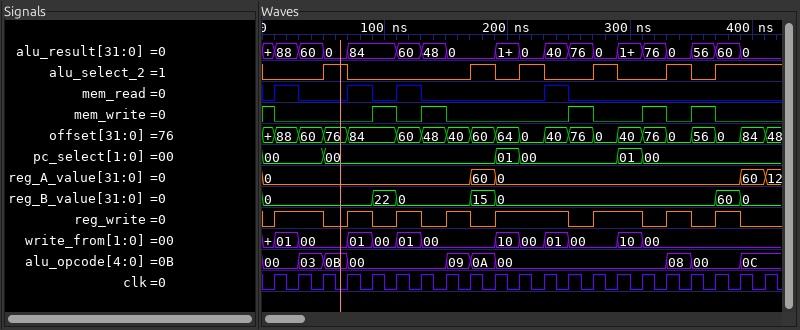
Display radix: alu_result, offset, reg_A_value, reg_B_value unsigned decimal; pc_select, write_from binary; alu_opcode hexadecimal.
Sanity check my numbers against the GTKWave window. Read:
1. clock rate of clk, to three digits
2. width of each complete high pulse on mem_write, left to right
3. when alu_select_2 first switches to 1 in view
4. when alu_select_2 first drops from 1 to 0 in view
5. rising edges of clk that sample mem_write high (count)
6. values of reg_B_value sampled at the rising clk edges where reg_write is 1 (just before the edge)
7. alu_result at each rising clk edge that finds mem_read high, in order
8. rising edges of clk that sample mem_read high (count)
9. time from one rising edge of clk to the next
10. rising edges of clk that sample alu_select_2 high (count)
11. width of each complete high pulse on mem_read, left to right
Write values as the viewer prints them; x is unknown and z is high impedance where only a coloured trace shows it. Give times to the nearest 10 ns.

50.0 MHz
20 ns, 20 ns, 20 ns, 20 ns, 20 ns
50 ns
70 ns
6
0, 0, 0, 0, 0, 0, 0, 0, 0, 0, 0, 60
88, 84, 60, 40
4
20 ns
7
20 ns, 20 ns, 20 ns, 20 ns
